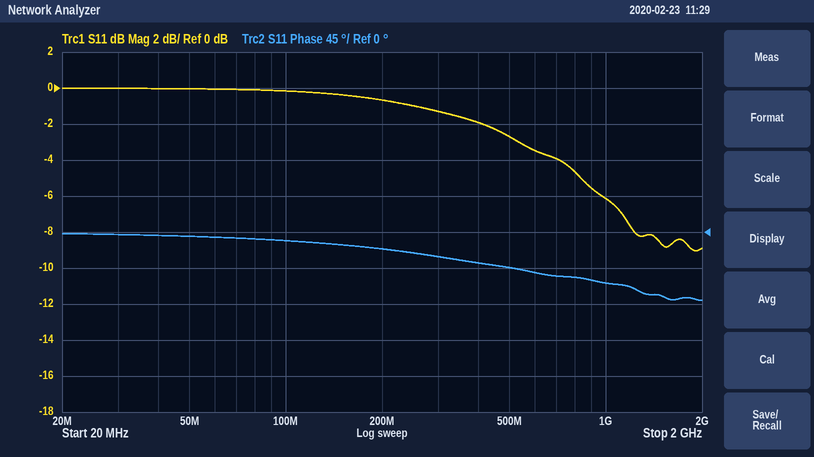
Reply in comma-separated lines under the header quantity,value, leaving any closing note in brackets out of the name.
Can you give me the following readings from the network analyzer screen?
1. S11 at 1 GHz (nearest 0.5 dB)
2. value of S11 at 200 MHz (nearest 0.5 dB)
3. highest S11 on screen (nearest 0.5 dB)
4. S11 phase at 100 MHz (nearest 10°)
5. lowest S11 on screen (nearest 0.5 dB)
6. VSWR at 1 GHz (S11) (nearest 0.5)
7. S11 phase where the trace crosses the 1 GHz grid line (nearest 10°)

quantity,value
S11 at 1 GHz,-6.0 dB
value of S11 at 200 MHz,-0.5 dB
highest S11 on screen,0.0 dB
S11 phase at 100 MHz,-10°
lowest S11 on screen,-9.0 dB
VSWR at 1 GHz (S11),3.0
S11 phase where the trace crosses the 1 GHz grid line,-60°
